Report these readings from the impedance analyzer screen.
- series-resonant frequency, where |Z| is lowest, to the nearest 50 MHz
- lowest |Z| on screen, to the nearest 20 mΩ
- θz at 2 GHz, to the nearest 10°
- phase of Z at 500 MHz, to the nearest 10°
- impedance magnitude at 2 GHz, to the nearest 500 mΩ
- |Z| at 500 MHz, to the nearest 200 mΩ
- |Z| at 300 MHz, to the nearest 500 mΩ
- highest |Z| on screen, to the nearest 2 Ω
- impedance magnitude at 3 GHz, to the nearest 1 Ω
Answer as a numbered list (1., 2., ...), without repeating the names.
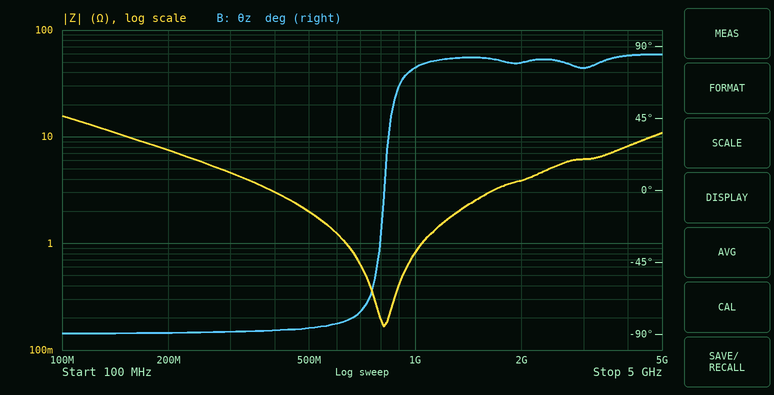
1. 800 MHz
2. 160 mΩ
3. 80°
4. -90°
5. 4.0 Ω
6. 2.0 Ω
7. 4.5 Ω
8. 16 Ω
9. 6 Ω
